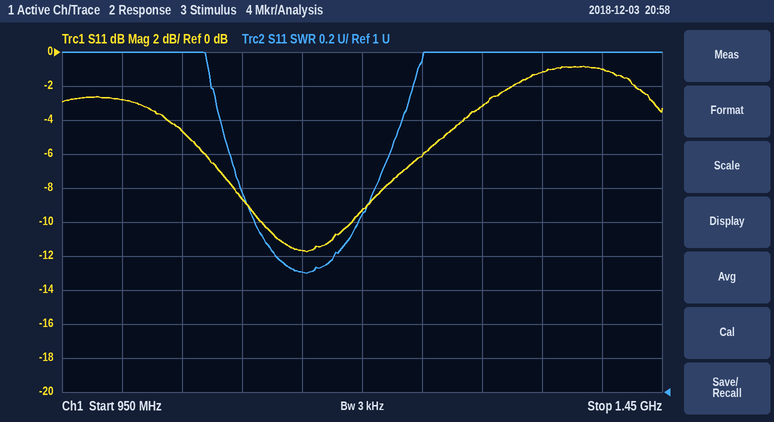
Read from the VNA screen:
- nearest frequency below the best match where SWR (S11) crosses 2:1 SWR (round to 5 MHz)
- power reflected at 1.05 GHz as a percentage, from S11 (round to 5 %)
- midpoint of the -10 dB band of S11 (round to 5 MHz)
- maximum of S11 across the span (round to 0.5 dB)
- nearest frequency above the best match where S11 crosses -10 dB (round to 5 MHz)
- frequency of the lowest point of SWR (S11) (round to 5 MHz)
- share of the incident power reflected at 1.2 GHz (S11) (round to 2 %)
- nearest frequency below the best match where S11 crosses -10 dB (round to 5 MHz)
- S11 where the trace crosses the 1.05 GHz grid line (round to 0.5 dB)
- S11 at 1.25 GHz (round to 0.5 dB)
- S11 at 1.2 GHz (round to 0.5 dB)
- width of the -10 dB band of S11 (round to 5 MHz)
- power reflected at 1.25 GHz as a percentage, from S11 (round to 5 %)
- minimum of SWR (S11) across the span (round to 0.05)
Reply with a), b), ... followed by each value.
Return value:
a) 1.110 GHz
b) 35 %
c) 1.155 GHz
d) -1.0 dB
e) 1.190 GHz
f) 1.155 GHz
g) 12 %
h) 1.115 GHz
i) -4.5 dB
j) -6.0 dB
k) -9.5 dB
l) 75 MHz
m) 25 %
n) 1.70
